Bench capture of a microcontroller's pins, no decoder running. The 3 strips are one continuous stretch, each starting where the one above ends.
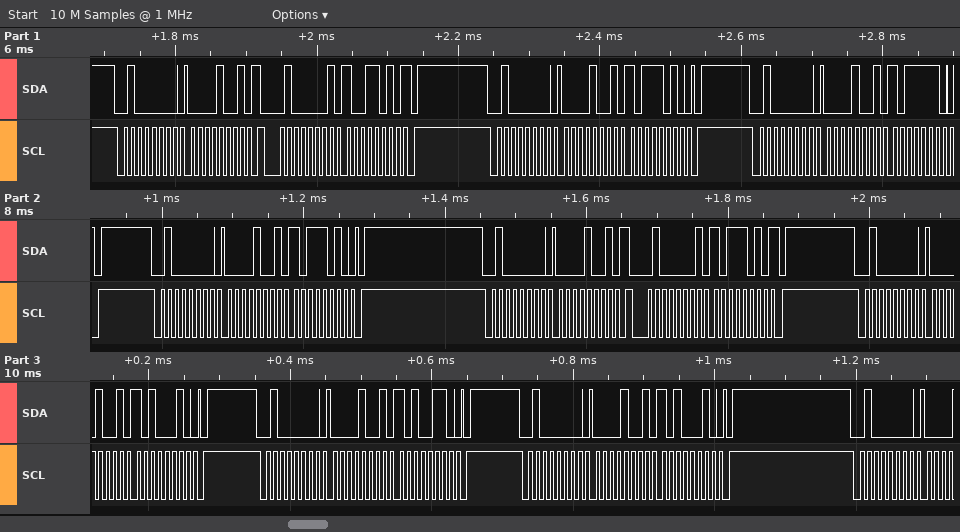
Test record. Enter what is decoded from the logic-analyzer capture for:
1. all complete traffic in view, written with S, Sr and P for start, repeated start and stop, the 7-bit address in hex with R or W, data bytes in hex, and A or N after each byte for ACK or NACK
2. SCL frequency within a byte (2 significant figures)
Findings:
S 20W A 09 A Sr 20R A 9A N P S 20W A 09 A BA A P S 20W A 09 A BE A P S 20W A 09 A BA A P S 20W A 09 A Sr 20R A BA N P S 20W A 09 A A2 A P S 20W A 09 A A6 A P S 20W A 09 A A2 A P S 20W A
100 kHz
